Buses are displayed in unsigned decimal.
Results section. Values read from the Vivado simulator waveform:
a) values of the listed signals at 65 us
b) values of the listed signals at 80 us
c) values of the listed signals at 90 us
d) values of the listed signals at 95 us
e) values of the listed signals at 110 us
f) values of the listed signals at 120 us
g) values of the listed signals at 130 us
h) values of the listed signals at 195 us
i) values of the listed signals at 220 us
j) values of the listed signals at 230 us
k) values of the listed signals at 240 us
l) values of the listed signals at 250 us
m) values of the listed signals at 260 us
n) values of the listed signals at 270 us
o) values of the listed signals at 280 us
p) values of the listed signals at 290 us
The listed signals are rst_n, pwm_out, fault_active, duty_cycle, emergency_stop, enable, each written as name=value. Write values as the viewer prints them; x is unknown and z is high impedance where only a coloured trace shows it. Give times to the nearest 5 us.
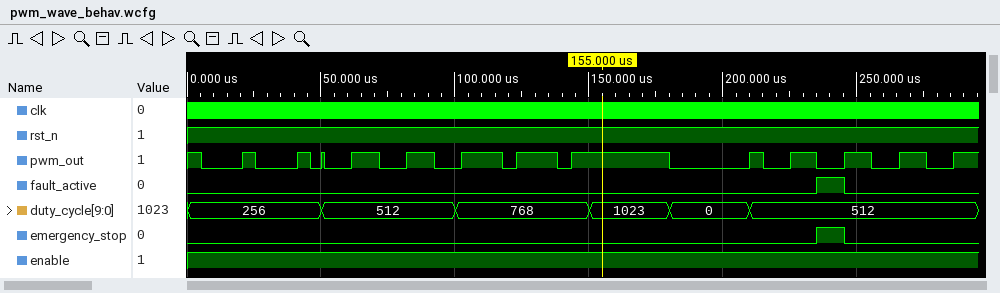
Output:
rst_n=1, pwm_out=1, fault_active=0, duty_cycle=512, emergency_stop=0, enable=1
rst_n=1, pwm_out=0, fault_active=0, duty_cycle=512, emergency_stop=0, enable=1
rst_n=1, pwm_out=1, fault_active=0, duty_cycle=512, emergency_stop=0, enable=1
rst_n=1, pwm_out=0, fault_active=0, duty_cycle=512, emergency_stop=0, enable=1
rst_n=1, pwm_out=1, fault_active=0, duty_cycle=768, emergency_stop=0, enable=1
rst_n=1, pwm_out=0, fault_active=0, duty_cycle=768, emergency_stop=0, enable=1
rst_n=1, pwm_out=1, fault_active=0, duty_cycle=768, emergency_stop=0, enable=1
rst_n=1, pwm_out=0, fault_active=0, duty_cycle=0, emergency_stop=0, enable=1
rst_n=1, pwm_out=0, fault_active=0, duty_cycle=512, emergency_stop=0, enable=1
rst_n=1, pwm_out=1, fault_active=0, duty_cycle=512, emergency_stop=0, enable=1
rst_n=1, pwm_out=0, fault_active=1, duty_cycle=512, emergency_stop=1, enable=1
rst_n=1, pwm_out=1, fault_active=0, duty_cycle=512, emergency_stop=0, enable=1
rst_n=1, pwm_out=0, fault_active=0, duty_cycle=512, emergency_stop=0, enable=1
rst_n=1, pwm_out=1, fault_active=0, duty_cycle=512, emergency_stop=0, enable=1
rst_n=1, pwm_out=0, fault_active=0, duty_cycle=512, emergency_stop=0, enable=1
rst_n=1, pwm_out=1, fault_active=0, duty_cycle=512, emergency_stop=0, enable=1
